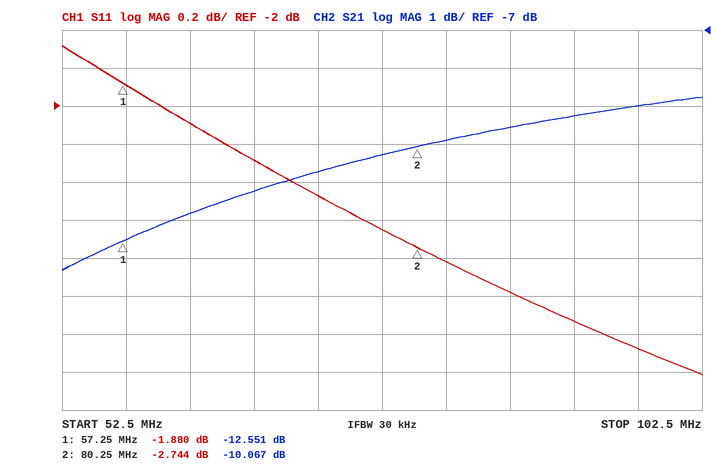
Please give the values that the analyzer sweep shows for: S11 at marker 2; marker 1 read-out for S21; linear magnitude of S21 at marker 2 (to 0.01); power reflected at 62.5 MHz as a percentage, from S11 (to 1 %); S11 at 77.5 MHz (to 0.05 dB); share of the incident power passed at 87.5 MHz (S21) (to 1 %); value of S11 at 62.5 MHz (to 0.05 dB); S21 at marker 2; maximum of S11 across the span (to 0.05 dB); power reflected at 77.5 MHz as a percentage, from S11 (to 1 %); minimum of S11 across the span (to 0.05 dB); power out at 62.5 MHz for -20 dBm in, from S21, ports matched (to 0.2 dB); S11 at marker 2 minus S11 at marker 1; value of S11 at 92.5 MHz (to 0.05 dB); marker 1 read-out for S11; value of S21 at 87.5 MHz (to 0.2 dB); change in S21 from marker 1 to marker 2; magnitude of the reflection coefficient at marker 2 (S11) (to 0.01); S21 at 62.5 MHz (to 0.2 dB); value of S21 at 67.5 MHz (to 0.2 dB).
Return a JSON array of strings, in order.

["-2.744 dB", "-12.551 dB", "0.31", "62 %", "-2.65 dB", "11 %", "-2.10 dB", "-10.067 dB", "-1.70 dB", "54 %", "-3.40 dB", "-31.8 dBm", "-0.864 dB", "-3.15 dB", "-1.880 dB", "-9.6 dB", "2.484 dB", "0.73", "-11.8 dB", "-11.2 dB"]
